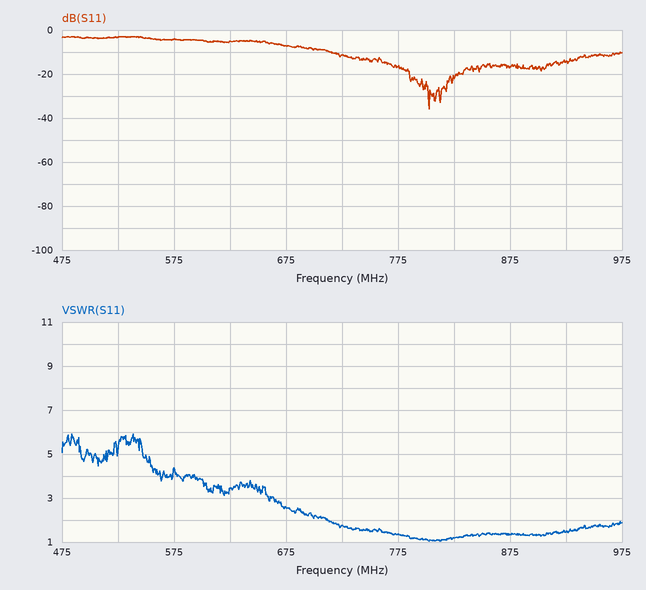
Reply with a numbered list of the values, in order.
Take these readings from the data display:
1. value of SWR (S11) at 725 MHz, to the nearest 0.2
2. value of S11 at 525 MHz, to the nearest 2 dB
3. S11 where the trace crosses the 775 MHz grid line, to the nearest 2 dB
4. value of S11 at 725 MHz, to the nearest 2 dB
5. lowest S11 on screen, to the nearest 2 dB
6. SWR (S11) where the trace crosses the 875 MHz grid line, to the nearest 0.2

1. 1.8
2. -4 dB
3. -16 dB
4. -12 dB
5. -36 dB
6. 1.4
